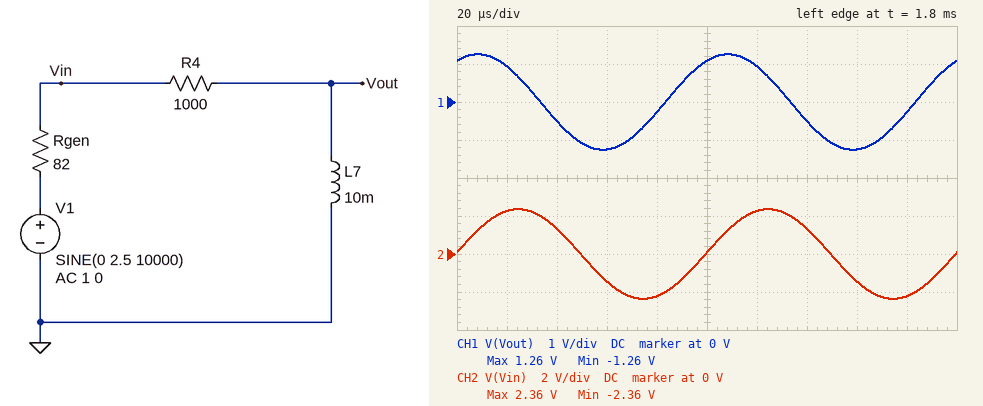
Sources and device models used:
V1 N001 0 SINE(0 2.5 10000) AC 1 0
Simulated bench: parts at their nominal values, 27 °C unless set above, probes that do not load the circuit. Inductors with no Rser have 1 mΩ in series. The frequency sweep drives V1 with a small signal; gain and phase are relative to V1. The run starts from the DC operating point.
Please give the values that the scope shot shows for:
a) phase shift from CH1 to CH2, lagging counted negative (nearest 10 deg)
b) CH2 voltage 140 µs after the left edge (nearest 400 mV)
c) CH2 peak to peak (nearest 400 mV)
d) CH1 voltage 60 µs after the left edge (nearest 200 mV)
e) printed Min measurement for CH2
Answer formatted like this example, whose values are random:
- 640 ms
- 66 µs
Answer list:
- -60 deg
- 1.2 V
- 4.8 V
- -1.2 V
- -2.36 V
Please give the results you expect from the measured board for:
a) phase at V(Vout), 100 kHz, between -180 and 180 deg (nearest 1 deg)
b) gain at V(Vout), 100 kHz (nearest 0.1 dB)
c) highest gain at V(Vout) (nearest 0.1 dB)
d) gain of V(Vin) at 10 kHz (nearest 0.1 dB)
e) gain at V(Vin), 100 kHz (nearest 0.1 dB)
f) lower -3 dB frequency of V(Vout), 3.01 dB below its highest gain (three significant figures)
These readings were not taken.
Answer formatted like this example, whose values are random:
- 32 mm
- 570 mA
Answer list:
- 10 deg
- -0.1 dB
- 0 dB
- -0.5 dB
- 0 dB
- 17.2 kHz
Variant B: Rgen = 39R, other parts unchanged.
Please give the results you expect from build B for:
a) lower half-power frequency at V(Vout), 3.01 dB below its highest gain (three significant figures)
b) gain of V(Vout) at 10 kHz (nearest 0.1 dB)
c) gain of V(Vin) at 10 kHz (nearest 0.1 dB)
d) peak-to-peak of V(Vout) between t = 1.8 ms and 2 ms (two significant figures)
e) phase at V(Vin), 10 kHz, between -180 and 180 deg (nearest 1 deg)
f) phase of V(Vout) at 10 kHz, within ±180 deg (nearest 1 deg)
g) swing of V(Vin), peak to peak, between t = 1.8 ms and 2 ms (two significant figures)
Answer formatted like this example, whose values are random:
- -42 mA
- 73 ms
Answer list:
- 16.5 kHz
- -5.7 dB
- -0.2 dB
- 2.6 V
- 1 deg
- 59 deg
- 4.9 V
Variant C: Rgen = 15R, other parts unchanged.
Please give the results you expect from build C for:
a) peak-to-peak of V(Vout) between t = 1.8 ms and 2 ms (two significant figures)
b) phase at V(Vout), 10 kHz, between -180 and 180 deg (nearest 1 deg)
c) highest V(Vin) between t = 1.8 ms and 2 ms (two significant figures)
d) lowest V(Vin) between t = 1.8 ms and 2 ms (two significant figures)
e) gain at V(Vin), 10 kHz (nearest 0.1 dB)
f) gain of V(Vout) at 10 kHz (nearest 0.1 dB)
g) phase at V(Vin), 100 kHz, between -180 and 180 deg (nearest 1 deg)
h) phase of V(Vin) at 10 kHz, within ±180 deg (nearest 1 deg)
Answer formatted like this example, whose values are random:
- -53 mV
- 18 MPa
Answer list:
- 2.6 V
- 58 deg
- 2.5 V
- -2.5 V
- -0.1 dB
- -5.6 dB
- 0 deg
- 0 deg
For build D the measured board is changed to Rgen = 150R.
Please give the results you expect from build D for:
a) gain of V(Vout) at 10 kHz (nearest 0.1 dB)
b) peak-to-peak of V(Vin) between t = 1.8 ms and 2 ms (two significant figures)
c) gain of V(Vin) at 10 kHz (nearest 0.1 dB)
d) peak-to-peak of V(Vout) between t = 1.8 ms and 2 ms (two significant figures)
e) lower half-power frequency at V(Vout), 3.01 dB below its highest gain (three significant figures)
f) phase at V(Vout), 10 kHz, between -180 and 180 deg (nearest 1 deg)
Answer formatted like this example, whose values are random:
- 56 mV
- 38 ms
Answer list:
- -6.4 dB
- 4.5 V
- -0.9 dB
- 2.4 V
- 18.3 kHz
- 61 deg
